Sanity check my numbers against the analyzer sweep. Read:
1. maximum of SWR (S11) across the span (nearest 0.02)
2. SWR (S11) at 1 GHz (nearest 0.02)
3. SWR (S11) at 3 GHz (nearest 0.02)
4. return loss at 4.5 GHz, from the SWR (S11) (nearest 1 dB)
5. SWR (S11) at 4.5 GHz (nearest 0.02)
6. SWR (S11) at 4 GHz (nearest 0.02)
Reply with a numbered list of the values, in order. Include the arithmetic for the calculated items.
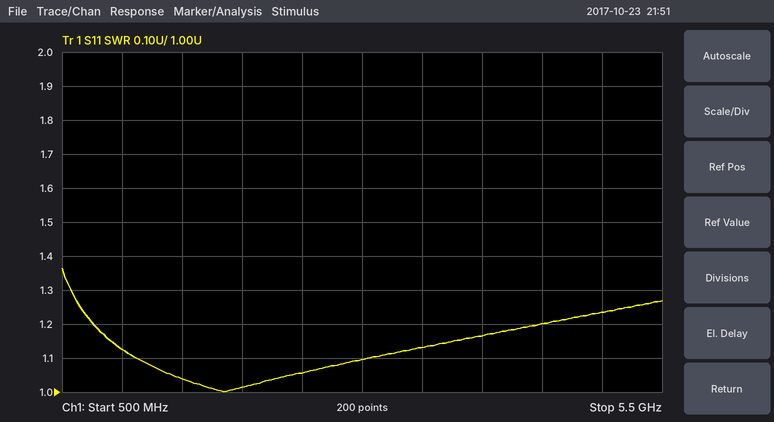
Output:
1. 1.36
2. 1.12
3. 1.10
4. −20 log10((1.2 − 1)/(1.2 + 1)) ≈ 21 dB
5. 1.20
6. 1.16
